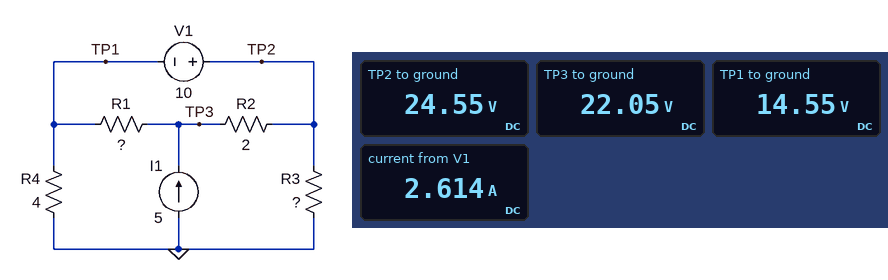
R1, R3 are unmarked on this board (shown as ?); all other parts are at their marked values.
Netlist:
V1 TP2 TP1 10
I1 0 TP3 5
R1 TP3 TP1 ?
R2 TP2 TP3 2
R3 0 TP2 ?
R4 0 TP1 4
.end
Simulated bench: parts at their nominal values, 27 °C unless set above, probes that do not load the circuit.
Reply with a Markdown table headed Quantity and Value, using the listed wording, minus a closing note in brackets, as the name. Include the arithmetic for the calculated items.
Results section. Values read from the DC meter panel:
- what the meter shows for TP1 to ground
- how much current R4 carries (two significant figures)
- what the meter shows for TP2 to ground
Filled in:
| Quantity | Value |
|---|---|
| what the meter shows for TP1 to ground | 14.55 V |
| how much current R4 carries | (14.55 V) / 4 Ω = 3.6 A |
| what the meter shows for TP2 to ground | 24.55 V |
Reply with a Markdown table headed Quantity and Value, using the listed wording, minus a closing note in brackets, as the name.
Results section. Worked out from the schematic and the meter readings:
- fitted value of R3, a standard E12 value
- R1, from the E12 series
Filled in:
| Quantity | Value |
|---|---|
| fitted value of R3, a standard E12 value | 18 Ω |
| R1, from the E12 series | 1.2 Ω |
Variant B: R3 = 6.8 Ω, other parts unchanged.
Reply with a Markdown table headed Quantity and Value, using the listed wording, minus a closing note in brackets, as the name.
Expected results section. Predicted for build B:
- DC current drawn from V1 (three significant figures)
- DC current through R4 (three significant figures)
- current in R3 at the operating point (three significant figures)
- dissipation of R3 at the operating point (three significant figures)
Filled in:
| Quantity | Value |
|---|---|
| DC current drawn from V1 | 4.03 A |
| DC current through R4 | 2.22 A |
| current in R3 at the operating point | 2.78 A |
| dissipation of R3 at the operating point | 52.5 W |
